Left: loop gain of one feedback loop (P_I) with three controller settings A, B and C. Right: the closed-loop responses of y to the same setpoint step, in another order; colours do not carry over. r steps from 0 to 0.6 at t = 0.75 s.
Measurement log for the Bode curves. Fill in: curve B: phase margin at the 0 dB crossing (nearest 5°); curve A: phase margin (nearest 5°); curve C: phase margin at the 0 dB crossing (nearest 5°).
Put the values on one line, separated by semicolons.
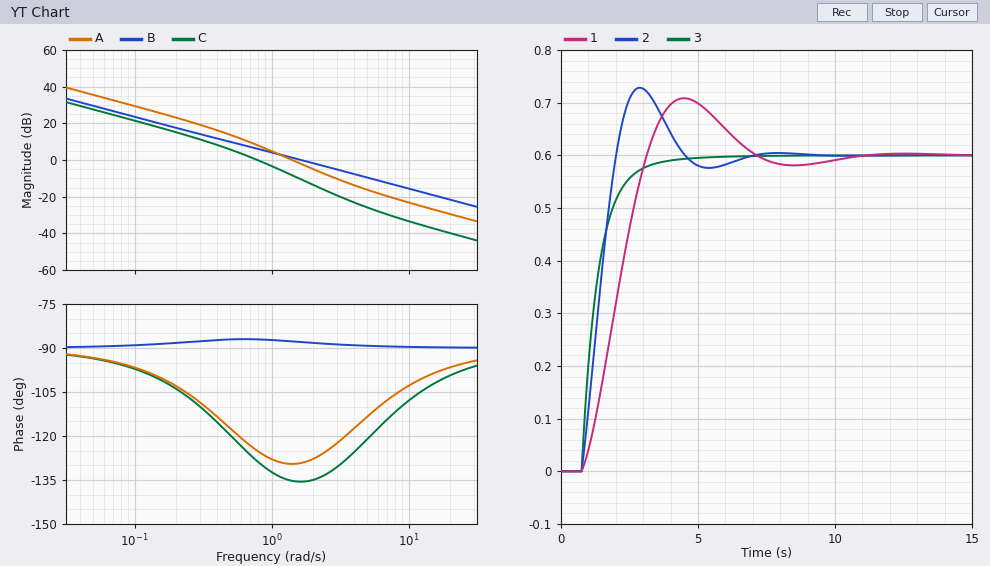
90°; 50°; 50°
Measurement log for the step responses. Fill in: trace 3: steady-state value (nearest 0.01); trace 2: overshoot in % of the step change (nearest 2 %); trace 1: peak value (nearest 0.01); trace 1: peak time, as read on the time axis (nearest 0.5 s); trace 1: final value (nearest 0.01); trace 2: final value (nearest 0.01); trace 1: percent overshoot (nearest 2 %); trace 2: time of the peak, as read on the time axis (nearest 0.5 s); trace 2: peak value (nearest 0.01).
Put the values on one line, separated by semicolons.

0.60; 22 %; 0.71; 4.5 s; 0.60; 0.60; 18 %; 3.0 s; 0.73
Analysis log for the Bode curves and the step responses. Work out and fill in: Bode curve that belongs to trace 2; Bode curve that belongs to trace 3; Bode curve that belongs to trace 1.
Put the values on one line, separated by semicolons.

A; B; C
